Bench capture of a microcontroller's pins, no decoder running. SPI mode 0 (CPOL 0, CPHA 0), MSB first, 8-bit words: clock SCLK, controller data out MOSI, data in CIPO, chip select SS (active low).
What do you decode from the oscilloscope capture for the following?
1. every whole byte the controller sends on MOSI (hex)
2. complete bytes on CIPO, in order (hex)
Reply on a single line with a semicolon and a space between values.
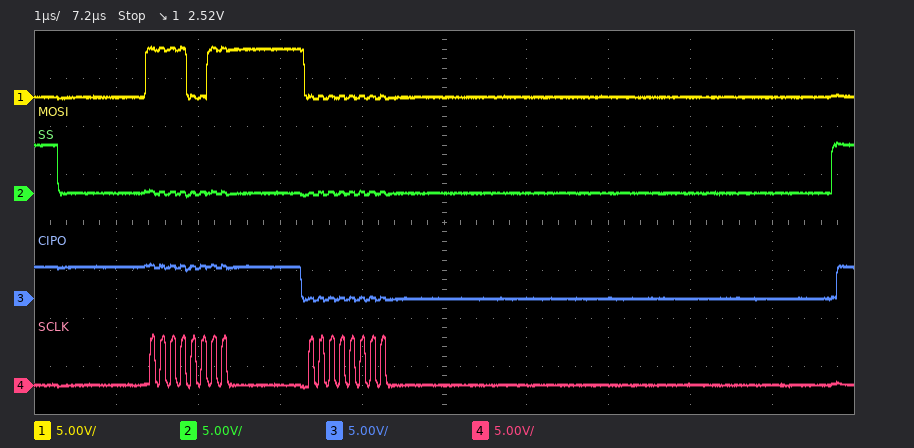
0xF3 0x00; 0xFF 0x00
